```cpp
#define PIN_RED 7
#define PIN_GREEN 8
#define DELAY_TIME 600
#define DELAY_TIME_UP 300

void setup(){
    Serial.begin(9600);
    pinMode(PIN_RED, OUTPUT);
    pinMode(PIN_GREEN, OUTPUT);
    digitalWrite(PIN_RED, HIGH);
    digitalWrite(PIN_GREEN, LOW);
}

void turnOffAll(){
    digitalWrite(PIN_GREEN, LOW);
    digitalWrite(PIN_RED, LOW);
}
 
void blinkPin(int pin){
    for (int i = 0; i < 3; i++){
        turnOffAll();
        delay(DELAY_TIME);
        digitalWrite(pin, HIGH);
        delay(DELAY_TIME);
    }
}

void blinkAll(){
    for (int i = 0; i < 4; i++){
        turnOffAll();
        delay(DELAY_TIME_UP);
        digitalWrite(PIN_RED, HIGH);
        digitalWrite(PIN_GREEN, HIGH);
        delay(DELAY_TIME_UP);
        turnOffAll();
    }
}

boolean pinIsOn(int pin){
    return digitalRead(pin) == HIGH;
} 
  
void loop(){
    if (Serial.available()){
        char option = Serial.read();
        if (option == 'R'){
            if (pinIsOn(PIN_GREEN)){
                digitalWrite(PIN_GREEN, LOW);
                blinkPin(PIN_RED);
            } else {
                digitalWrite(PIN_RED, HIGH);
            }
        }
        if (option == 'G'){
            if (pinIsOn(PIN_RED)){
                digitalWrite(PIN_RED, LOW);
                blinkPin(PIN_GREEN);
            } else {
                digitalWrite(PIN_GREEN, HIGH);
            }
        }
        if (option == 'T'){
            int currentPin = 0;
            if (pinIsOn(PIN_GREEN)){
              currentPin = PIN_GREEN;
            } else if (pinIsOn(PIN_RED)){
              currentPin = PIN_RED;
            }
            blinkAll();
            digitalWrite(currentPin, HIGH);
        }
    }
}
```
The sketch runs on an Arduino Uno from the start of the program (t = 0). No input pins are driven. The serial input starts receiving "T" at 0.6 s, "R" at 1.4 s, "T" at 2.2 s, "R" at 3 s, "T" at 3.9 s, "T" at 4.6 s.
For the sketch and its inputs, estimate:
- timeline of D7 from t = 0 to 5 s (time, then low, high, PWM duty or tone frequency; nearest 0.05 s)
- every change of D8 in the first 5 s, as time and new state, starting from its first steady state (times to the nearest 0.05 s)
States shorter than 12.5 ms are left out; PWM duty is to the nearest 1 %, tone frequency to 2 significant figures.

0 s high; 0.6 s low; 0.9 s high; 1.2 s low; 1.5 s high; 1.8 s low; 2.1 s high; 2.4 s low; 2.7 s high; 3 s low; 3.3 s high; 3.6 s low; 3.9 s high; 4.2 s low; 4.5 s high; 4.8 s low
0 s low; 0.9 s high; 1.2 s low; 1.5 s high; 1.8 s low; 2.1 s high; 2.4 s low; 2.7 s high; 3 s low; 3.3 s high; 3.6 s low; 3.9 s high; 4.2 s low; 4.5 s high; 4.8 s low
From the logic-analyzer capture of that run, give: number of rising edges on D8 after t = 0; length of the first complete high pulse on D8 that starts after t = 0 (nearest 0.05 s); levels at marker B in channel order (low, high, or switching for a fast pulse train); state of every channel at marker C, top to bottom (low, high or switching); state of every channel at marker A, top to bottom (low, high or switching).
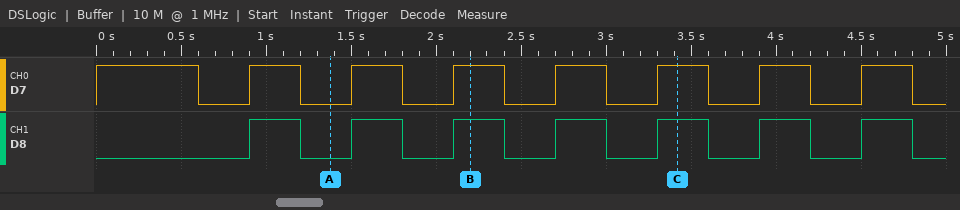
7
0.30 s
D7 high, D8 high
D7 high, D8 high
D7 low, D8 low
